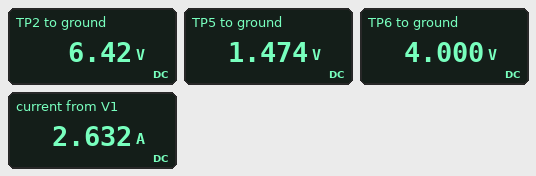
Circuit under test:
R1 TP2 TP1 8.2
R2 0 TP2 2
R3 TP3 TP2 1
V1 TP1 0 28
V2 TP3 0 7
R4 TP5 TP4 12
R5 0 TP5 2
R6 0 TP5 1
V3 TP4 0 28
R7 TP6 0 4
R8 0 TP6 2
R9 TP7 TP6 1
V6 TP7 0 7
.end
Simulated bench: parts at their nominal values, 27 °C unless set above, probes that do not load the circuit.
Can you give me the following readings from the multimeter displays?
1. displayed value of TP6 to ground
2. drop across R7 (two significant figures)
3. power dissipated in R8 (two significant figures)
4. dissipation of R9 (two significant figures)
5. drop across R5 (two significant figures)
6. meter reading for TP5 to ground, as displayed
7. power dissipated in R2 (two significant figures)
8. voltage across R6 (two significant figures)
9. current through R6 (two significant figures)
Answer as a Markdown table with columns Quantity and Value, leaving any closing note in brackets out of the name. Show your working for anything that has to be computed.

| Quantity | Value |
|---|---|
| displayed value of TP6 to ground | 4.000 V |
| drop across R7 | 4 V = 4.0 V |
| power dissipated in R8 | (4 V)^2 / 2 Ω = 8.0 W |
| dissipation of R9 | (7 V - 4 V)^2 / 1 Ω = 9.0 W |
| drop across R5 | 1.474 V = 1.5 V |
| meter reading for TP5 to ground, as displayed | 1.474 V |
| power dissipated in R2 | (6.42 V)^2 / 2 Ω = 21 W |
| voltage across R6 | 1.474 V = 1.5 V |
| current through R6 | (1.474 V) / 1 Ω = 1.5 A |
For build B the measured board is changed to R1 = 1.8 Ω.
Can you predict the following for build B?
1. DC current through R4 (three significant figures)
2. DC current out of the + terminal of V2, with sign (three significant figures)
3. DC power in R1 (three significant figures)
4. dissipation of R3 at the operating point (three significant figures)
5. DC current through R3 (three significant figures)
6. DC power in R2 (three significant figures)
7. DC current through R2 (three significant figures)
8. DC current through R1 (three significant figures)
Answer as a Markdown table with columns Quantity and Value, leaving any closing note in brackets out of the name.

| Quantity | Value |
|---|---|
| DC current through R4 | 2.21 A |
| DC current out of the + terminal of V2, with sign | -3.97 A |
| DC power in R1 | 161 W |
| dissipation of R3 at the operating point | 15.8 W |
| DC current through R3 | 3.97 A |
| DC power in R2 | 60.2 W |
| DC current through R2 | 5.49 A |
| DC current through R1 | 9.46 A |
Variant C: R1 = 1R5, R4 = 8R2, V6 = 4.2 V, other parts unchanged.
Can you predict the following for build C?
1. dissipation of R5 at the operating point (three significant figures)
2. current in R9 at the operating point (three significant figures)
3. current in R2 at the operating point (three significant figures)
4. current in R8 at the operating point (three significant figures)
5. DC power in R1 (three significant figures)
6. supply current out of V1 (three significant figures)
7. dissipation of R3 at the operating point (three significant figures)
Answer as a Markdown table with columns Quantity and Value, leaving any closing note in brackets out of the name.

| Quantity | Value |
|---|---|
| dissipation of R5 at the operating point | 2.22 W |
| current in R9 at the operating point | 1.80 A |
| current in R2 at the operating point | 5.92 A |
| current in R8 at the operating point | 1.20 A |
| DC power in R1 | 174 W |
| supply current out of V1 | 10.8 A |
| dissipation of R3 at the operating point | 23.5 W |
